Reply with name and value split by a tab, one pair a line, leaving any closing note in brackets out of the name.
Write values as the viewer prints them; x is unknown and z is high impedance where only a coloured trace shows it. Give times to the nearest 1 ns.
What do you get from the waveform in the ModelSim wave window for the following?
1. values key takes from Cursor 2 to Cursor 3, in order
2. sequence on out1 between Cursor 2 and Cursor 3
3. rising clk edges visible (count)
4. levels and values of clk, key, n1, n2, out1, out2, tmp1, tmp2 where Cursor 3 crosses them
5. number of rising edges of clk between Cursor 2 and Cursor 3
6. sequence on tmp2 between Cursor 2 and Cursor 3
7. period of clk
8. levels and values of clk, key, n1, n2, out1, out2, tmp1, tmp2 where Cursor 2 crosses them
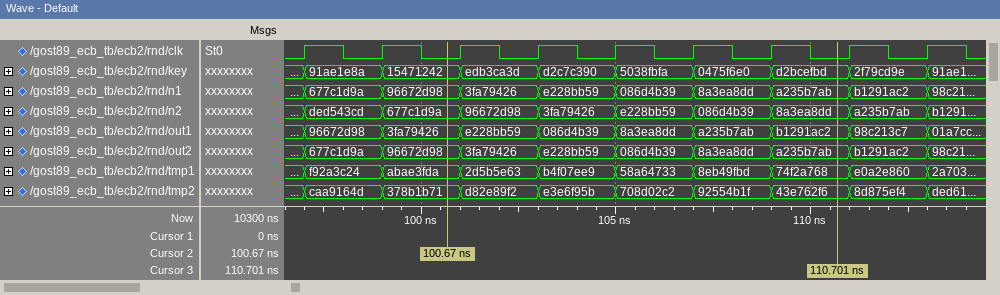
values key takes from Cursor 2 to Cursor 3, in order	15471242, edb3ca3d, d2c7c390, 5038fbfa, 0475f6e0, d2bcefbd
sequence on out1 between Cursor 2 and Cursor 3	3fa79426, e228bb59, 086d4b39, 8a3ea8dd, a235b7ab, b1291ac2
rising clk edges visible	9
levels and values of clk, key, n1, n2, out1, out2, tmp1, tmp2 where Cursor 3 crosses them	clk=0, key=d2bcefbd, n1=a235b7ab, n2=8a3ea8dd, out1=b1291ac2, out2=a235b7ab, tmp1=74f2a768, tmp2=43e762f6
number of rising edges of clk between Cursor 2 and Cursor 3	5
sequence on tmp2 between Cursor 2 and Cursor 3	378b1b71, d82e89f2, e3e6f95b, 708d02c2, 92554b1f, 43e762f6
period of clk	2 ns
levels and values of clk, key, n1, n2, out1, out2, tmp1, tmp2 where Cursor 2 crosses them	clk=0, key=15471242, n1=96672d98, n2=677c1d9a, out1=3fa79426, out2=96672d98, tmp1=abae3fda, tmp2=378b1b71
